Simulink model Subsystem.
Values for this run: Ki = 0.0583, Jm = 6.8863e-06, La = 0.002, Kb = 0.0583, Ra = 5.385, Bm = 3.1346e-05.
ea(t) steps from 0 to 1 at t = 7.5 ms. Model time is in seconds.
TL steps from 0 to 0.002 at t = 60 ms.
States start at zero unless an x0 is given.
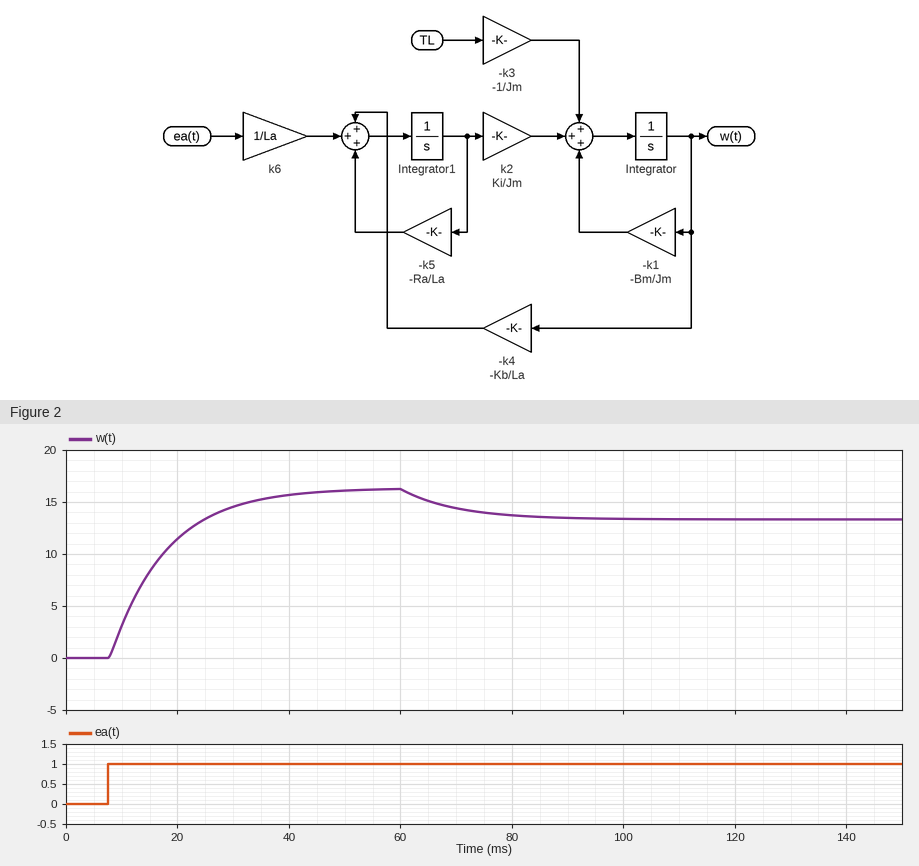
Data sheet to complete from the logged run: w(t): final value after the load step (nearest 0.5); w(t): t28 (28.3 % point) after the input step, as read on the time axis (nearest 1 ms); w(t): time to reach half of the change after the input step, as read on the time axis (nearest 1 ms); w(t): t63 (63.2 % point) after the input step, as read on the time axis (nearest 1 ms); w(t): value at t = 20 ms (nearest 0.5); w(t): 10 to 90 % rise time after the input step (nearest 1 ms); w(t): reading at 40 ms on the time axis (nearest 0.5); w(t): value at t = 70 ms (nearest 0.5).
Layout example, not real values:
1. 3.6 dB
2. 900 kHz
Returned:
1. 13.5
2. 11 ms
3. 15 ms
4. 18 ms
5. 11.5
6. 22 ms
7. 15.5
8. 14.5
